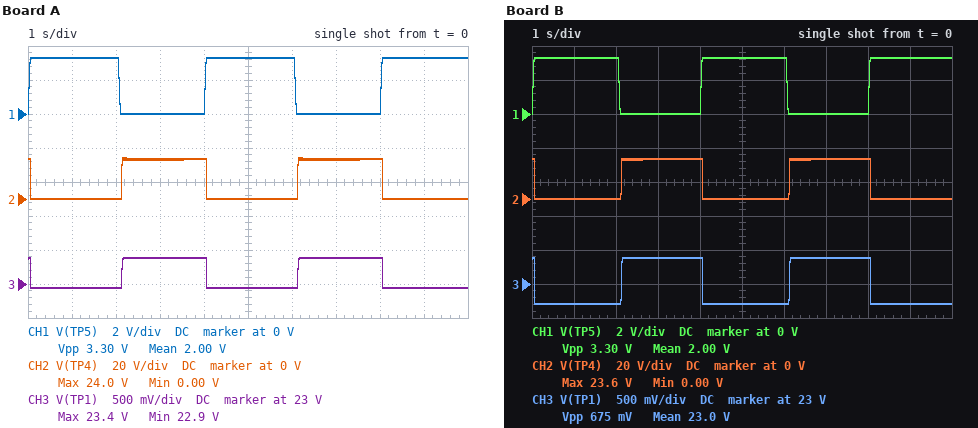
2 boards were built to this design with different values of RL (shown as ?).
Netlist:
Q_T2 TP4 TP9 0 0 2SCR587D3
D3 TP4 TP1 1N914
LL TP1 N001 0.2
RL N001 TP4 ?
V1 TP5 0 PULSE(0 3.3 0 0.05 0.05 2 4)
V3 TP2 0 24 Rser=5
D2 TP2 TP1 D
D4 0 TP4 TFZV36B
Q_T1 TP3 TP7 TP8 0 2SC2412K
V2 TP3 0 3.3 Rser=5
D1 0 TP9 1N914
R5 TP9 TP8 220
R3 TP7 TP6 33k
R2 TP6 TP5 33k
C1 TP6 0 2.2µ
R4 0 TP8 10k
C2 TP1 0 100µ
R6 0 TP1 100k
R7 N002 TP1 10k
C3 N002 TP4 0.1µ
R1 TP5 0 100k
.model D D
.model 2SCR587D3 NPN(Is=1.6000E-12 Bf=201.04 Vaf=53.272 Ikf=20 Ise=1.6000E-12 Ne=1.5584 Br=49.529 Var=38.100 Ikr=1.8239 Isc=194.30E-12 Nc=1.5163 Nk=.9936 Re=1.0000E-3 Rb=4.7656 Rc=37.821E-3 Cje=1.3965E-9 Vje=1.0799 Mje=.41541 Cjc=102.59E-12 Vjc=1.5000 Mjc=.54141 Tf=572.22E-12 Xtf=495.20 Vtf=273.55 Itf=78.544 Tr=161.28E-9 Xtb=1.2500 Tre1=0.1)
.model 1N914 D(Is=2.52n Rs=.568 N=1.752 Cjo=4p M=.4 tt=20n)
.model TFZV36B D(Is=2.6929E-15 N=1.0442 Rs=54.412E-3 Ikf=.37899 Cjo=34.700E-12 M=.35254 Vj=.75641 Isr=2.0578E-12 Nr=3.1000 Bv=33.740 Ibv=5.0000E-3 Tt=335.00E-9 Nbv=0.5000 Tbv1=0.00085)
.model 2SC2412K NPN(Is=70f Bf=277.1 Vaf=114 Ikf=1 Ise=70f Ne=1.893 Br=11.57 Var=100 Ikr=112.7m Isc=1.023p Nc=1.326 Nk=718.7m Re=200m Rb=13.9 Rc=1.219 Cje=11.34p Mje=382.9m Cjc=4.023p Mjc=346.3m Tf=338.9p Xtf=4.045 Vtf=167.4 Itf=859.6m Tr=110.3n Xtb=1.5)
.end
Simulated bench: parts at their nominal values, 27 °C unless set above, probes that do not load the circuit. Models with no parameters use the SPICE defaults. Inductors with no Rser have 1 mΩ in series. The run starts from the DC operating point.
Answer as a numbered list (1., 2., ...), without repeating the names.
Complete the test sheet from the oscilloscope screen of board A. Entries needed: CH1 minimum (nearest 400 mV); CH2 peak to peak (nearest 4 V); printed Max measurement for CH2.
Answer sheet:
1. 0 V
2. 24 V
3. 24.0 V
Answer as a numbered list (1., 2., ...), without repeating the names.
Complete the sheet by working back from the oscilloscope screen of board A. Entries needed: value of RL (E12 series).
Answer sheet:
1. 390 Ω
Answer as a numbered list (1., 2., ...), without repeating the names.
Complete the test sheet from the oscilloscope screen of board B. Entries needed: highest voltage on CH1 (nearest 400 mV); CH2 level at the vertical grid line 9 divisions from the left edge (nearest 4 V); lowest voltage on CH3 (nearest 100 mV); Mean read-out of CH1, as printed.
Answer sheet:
1. 3.2 V
2. 0 V
3. 22.7 V
4. 2.00 V
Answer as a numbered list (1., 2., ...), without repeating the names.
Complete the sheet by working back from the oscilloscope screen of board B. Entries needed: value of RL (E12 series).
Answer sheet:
1. 220 Ω
